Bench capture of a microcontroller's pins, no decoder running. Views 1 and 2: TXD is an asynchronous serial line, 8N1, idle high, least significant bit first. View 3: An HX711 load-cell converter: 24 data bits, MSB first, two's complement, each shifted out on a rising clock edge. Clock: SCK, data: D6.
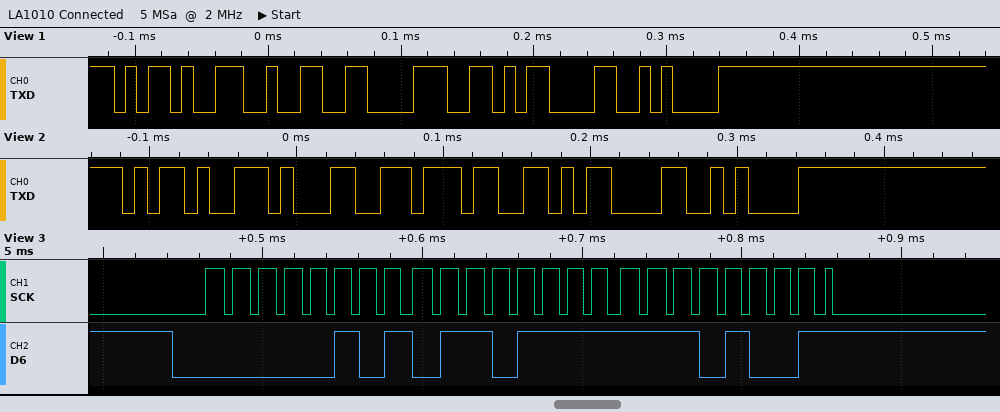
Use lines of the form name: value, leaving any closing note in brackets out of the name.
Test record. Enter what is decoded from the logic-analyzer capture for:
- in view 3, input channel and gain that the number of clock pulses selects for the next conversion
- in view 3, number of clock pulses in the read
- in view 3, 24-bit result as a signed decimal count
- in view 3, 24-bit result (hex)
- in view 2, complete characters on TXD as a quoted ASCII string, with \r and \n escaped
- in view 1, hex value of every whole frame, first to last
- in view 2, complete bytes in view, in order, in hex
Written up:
in view 3, input channel and gain that the number of clock pulses selects for the next conversion: channel A, gain 128
in view 3, number of clock pulses in the read: 25
in view 3, 24-bit result as a signed decimal count: 356329
in view 3, 24-bit result: 0x056FE9
in view 2, complete characters on TXD as a quoted ASCII string, with \r and \n escaped: "-17\r\n"
in view 1, hex value of every whole frame, first to last: 0x2D 0x32 0x38 0x0D 0x0A
in view 2, complete bytes in view, in order, in hex: 2D 31 37 0D 0A
